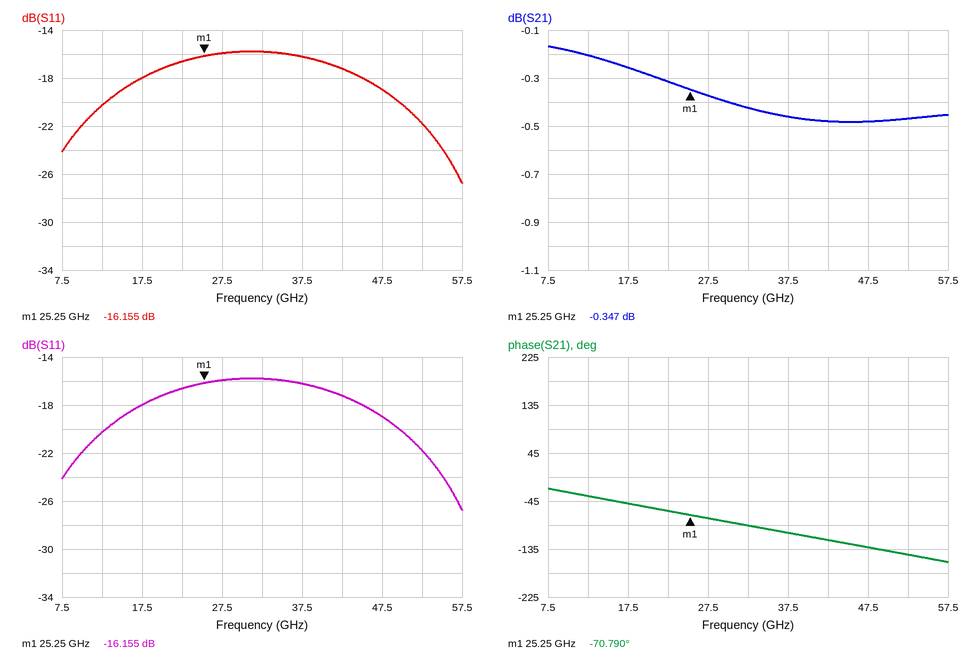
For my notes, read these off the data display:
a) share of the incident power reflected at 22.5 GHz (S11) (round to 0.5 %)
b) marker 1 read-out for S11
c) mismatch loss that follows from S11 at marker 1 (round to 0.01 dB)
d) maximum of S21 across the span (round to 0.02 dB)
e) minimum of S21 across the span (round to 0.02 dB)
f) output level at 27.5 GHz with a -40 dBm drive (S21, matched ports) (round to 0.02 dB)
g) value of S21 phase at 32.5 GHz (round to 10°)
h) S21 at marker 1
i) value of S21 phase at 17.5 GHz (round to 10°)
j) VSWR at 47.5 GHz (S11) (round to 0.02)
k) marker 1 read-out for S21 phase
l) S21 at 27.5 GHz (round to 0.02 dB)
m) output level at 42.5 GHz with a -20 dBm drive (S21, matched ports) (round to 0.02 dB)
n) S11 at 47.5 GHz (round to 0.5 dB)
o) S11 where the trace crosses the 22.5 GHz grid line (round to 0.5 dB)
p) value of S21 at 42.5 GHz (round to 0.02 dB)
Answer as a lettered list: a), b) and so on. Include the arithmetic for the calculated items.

a) 10^(-16.5/10) ≈ 2.24 %, so 2.0 % to the nearest 0.5 %
b) -16.155 dB
c) −10 log10(1 − 10^(-16.155/10)) ≈ 0.11 dB
d) -0.16 dB
e) -0.48 dB
f) -40 dBm + (-0.38 dB) = -40.38 dBm
g) -90°
h) -0.347 dB
i) -50°
j) |Γ| = 10^(-19/20) = 0.1122; VSWR = (1 + 0.1122)/(1 − 0.1122) ≈ 1.25, so 1.26 to the nearest 0.02
k) -70.790°
l) -0.38 dB
m) -20 dBm + (-0.48 dB) = -20.48 dBm
n) -19.0 dB
o) -16.5 dB
p) -0.48 dB
